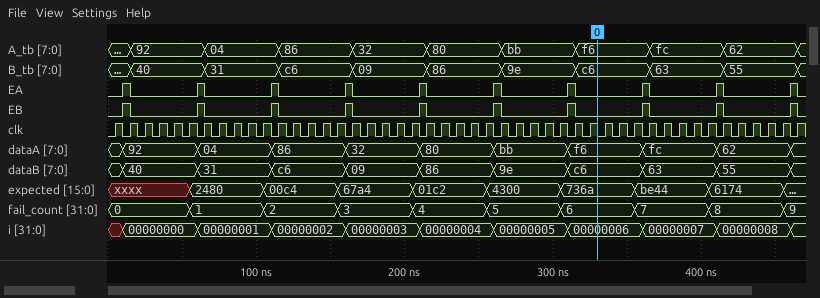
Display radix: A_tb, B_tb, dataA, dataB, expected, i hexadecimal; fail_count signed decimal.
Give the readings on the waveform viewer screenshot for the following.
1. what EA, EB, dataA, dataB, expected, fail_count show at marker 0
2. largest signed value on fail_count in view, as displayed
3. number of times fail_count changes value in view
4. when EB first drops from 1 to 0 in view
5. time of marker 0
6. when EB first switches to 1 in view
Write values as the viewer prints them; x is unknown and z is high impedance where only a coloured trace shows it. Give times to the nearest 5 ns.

EA=0, EB=0, dataA=f6, dataB=c6, expected=736a, fail_count=6
9
9
15 ns
330 ns
10 ns
